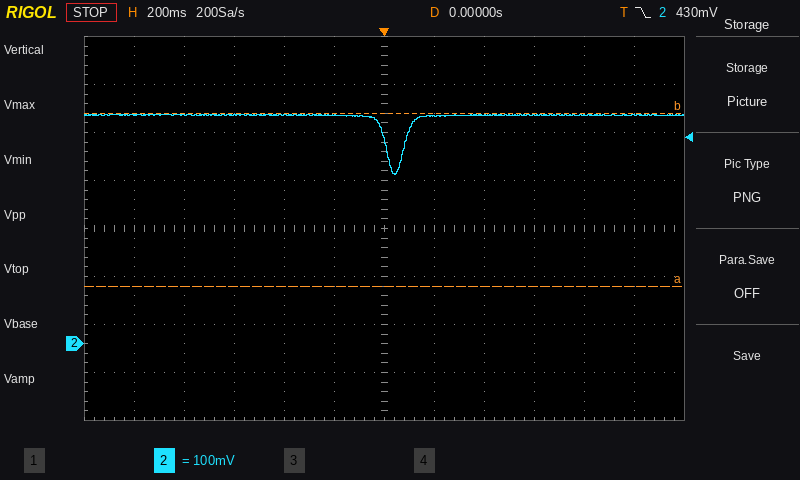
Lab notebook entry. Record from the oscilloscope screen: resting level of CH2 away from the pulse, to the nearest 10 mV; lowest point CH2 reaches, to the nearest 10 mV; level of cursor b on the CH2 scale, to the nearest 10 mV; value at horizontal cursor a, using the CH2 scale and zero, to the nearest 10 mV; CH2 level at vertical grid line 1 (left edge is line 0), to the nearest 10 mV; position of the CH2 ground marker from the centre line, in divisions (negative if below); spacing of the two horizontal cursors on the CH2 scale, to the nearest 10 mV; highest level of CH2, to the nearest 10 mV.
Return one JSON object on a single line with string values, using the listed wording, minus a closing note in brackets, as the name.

{"resting level of CH2 away from the pulse, to the nearest 10 mV": "480 mV", "lowest point CH2 reaches, to the nearest 10 mV": "350 mV", "level of cursor b on the CH2 scale, to the nearest 10 mV": "480 mV", "value at horizontal cursor a, using the CH2 scale and zero, to the nearest 10 mV": "120 mV", "CH2 level at vertical grid line 1 (left edge is line 0), to the nearest 10 mV": "480 mV", "position of the CH2 ground marker from the centre line, in divisions": "-2.4 div", "spacing of the two horizontal cursors on the CH2 scale, to the nearest 10 mV": "360 mV", "highest level of CH2, to the nearest 10 mV": "480 mV"}
